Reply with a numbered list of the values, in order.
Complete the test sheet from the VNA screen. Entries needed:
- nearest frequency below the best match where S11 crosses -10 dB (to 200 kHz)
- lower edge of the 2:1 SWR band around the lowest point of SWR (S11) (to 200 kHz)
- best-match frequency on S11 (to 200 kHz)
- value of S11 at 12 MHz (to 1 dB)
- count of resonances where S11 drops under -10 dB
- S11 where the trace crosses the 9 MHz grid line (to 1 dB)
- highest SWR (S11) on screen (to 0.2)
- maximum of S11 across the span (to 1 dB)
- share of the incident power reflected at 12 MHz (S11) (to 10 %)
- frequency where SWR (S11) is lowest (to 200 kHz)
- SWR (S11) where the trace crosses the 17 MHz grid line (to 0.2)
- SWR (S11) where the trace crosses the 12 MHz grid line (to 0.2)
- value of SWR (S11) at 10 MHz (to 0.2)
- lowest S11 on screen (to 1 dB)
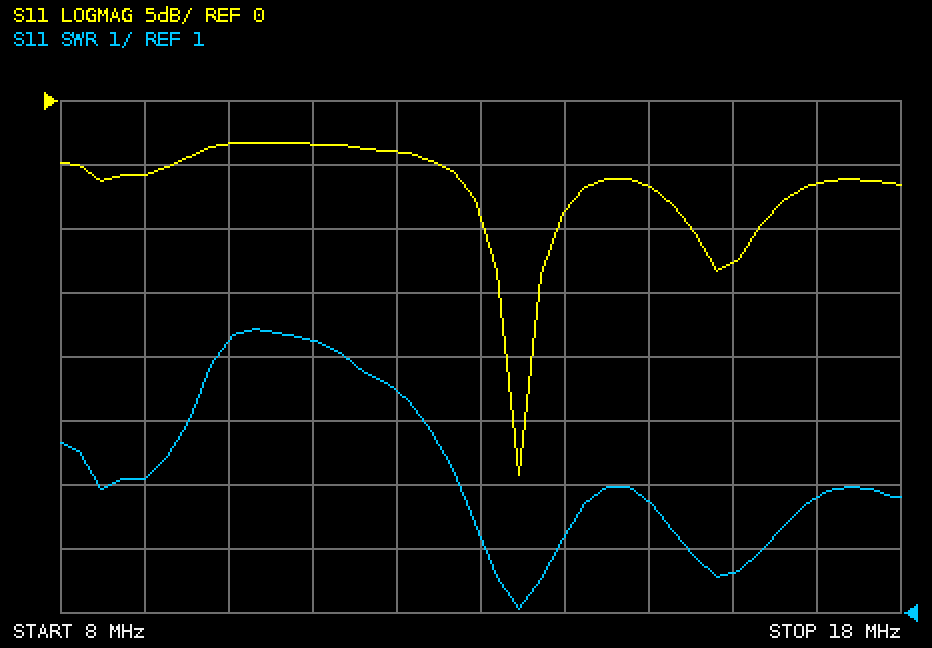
1. 13.0 MHz
2. 13.0 MHz
3. 13.4 MHz
4. -4 dB
5. 2
6. -6 dB
7. 5.4
8. -3 dB
9. 40 %
10. 13.4 MHz
11. 2.8
12. 4.4
13. 5.2
14. -29 dB
